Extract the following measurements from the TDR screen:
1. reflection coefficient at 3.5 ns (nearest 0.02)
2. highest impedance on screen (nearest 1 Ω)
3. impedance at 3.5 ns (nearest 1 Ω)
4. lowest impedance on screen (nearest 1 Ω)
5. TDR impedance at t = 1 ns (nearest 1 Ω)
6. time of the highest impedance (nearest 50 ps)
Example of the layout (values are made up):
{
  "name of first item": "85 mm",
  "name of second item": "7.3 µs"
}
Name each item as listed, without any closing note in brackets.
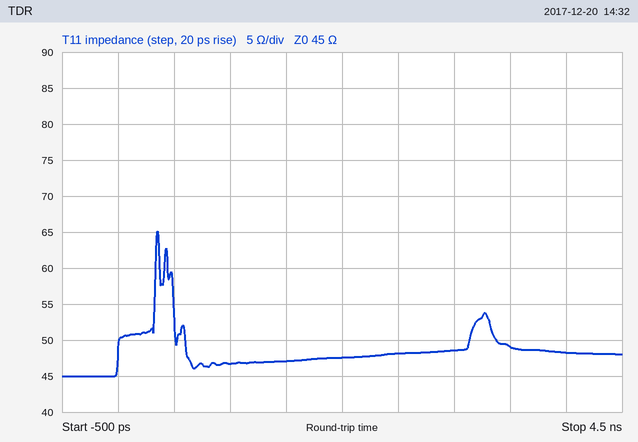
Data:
{
  "reflection coefficient at 3.5 ns": "+0.04",
  "highest impedance on screen": "65 Ω",
  "impedance at 3.5 ns": "49 Ω",
  "lowest impedance on screen": "45 Ω",
  "TDR impedance at t = 1 ns": "47 Ω",
  "time of the highest impedance": "350 ps"
}
